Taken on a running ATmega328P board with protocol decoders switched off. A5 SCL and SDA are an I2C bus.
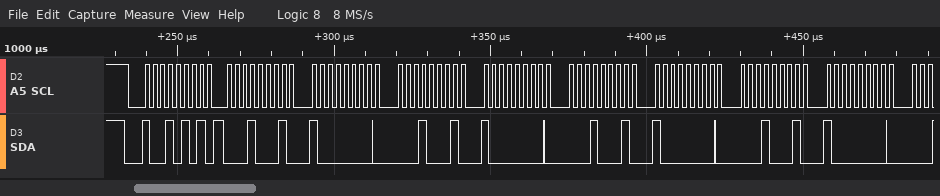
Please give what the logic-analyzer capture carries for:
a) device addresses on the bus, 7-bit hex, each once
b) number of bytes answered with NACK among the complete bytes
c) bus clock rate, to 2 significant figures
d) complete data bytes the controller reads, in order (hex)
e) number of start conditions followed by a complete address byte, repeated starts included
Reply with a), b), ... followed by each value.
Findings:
a) 0x4A
b) 0
c) 400 kHz
d) 11 80 11 80 11 80 11 80
e) 1
